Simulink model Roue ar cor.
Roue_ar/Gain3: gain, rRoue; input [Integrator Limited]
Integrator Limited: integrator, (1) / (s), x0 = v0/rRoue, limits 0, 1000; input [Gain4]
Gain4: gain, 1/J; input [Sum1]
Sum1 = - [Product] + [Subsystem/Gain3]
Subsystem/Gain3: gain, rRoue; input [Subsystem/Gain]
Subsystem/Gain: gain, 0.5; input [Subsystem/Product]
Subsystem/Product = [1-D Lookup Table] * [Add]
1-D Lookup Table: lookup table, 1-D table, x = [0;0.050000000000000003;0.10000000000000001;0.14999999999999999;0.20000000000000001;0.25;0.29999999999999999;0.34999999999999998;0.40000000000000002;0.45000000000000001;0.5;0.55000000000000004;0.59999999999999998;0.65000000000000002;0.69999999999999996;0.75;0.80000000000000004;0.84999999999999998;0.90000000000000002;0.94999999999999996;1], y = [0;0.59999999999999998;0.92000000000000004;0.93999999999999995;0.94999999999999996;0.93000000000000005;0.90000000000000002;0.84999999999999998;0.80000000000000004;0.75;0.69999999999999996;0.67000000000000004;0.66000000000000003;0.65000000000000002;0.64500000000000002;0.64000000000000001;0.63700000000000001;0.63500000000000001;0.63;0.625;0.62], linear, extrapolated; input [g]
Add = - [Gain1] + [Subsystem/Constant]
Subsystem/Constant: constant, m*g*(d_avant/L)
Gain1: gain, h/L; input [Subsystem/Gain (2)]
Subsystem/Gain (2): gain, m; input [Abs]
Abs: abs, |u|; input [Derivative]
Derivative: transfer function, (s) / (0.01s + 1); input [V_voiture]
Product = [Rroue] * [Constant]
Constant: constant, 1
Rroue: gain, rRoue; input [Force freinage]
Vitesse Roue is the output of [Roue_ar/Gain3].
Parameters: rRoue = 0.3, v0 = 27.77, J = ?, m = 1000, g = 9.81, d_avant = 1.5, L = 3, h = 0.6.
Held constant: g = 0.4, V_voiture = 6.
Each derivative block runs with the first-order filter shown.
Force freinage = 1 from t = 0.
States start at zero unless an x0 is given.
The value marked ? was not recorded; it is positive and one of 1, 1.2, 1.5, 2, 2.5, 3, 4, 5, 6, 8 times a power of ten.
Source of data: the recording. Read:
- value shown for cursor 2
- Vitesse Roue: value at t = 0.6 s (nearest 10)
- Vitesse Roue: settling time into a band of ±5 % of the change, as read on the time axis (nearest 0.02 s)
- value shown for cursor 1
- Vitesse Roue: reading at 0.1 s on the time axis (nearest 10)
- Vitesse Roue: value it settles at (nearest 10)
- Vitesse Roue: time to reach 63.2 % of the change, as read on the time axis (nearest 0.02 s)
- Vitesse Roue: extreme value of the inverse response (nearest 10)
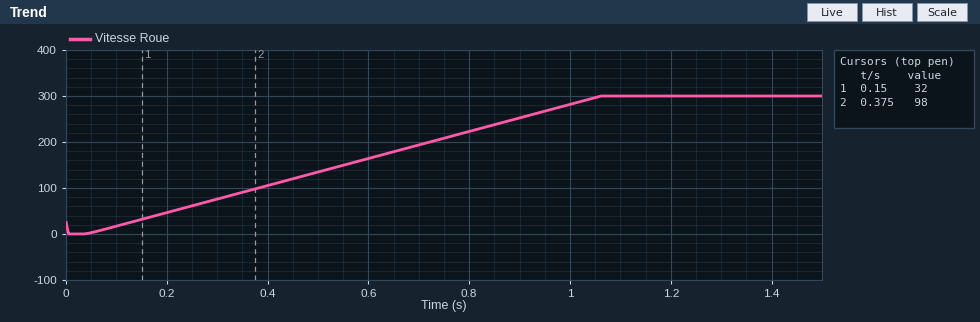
98
160
1.02 s
32
20
300
0.72 s
0
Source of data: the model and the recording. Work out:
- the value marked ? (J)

0.6
